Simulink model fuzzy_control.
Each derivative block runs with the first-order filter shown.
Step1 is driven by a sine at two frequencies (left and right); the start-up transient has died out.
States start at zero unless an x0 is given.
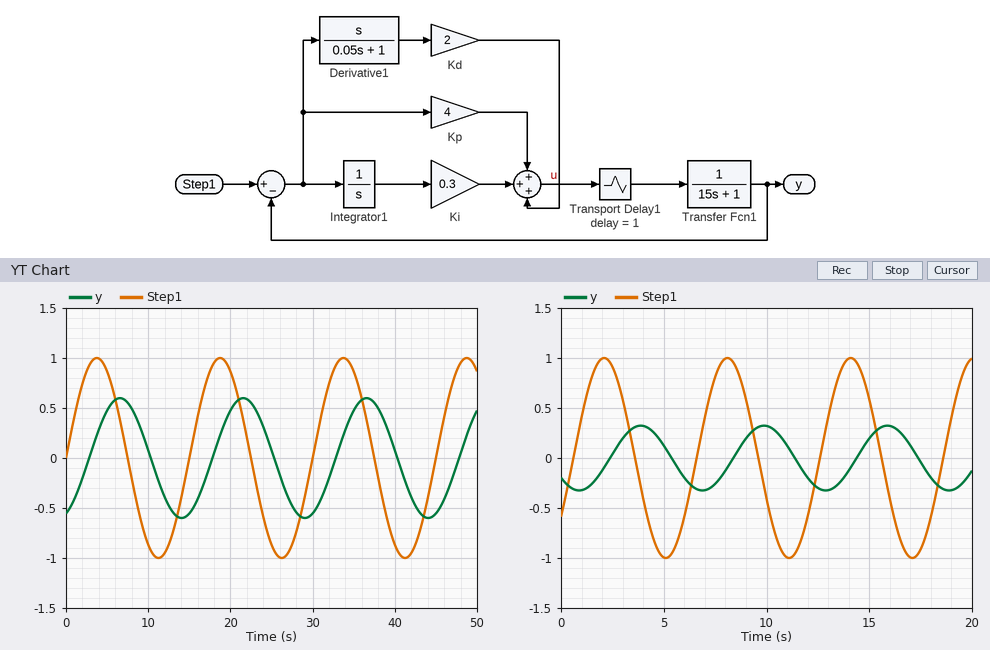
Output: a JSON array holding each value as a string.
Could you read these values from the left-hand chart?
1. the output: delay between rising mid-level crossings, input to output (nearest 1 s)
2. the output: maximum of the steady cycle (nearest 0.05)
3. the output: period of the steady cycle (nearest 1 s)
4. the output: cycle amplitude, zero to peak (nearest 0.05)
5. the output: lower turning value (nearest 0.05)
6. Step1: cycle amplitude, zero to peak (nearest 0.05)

["3 s", "0.60", "15 s", "0.60", "-0.60", "1.00"]
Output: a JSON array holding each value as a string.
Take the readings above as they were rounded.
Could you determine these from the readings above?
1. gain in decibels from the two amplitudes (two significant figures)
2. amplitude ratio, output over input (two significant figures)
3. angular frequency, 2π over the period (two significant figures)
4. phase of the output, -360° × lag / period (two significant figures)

["-4.4 dB", "0.60", "0.42 rad/s", "-72°"]
